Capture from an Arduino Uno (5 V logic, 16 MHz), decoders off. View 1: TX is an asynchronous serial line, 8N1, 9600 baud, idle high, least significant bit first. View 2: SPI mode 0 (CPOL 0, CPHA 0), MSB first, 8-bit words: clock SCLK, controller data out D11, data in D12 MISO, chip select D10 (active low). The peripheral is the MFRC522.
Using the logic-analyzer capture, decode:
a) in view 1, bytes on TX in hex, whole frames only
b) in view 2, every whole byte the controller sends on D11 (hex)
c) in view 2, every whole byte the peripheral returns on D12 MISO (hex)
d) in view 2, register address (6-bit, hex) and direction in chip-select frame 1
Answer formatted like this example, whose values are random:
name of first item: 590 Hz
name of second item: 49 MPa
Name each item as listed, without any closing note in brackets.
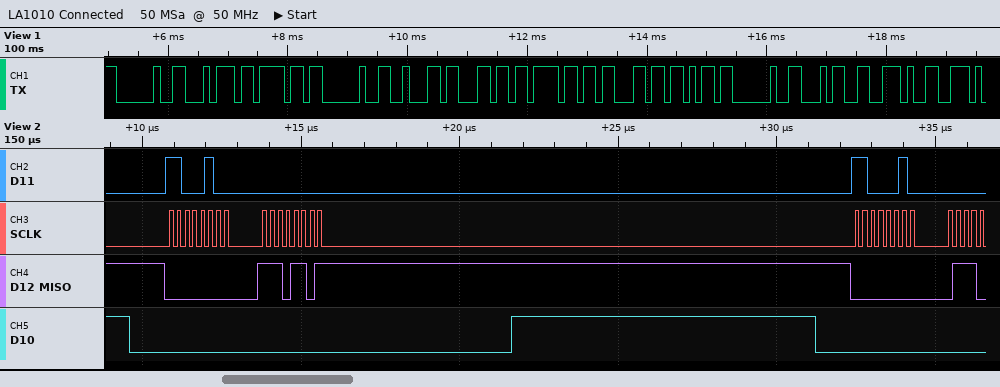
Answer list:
in view 1, bytes on TX in hex, whole frames only: 20 74 6F 20 62 6C 6F 63 6B 20 34 2E
in view 2, every whole byte the controller sends on D11: 0xC4 0x00 0xC2
in view 2, every whole byte the peripheral returns on D12 MISO: 0x00 0xED 0x00
in view 2, register address (6-bit, hex) and direction in chip-select frame 1: 0x22 read
